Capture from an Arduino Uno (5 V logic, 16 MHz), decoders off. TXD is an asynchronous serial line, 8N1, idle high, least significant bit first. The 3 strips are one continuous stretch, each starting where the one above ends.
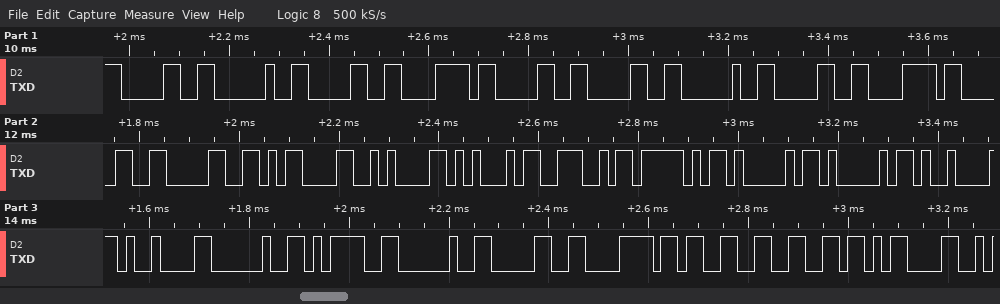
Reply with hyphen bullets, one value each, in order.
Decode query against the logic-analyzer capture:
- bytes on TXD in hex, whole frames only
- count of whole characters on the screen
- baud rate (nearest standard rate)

- 30 20 30 78 30 30 20 30 78 30 30 0D 0A 45 4E 5F 41 41 09 09 20 3D 20 30 78 33 66 0D
- 28
- 57600 baud
